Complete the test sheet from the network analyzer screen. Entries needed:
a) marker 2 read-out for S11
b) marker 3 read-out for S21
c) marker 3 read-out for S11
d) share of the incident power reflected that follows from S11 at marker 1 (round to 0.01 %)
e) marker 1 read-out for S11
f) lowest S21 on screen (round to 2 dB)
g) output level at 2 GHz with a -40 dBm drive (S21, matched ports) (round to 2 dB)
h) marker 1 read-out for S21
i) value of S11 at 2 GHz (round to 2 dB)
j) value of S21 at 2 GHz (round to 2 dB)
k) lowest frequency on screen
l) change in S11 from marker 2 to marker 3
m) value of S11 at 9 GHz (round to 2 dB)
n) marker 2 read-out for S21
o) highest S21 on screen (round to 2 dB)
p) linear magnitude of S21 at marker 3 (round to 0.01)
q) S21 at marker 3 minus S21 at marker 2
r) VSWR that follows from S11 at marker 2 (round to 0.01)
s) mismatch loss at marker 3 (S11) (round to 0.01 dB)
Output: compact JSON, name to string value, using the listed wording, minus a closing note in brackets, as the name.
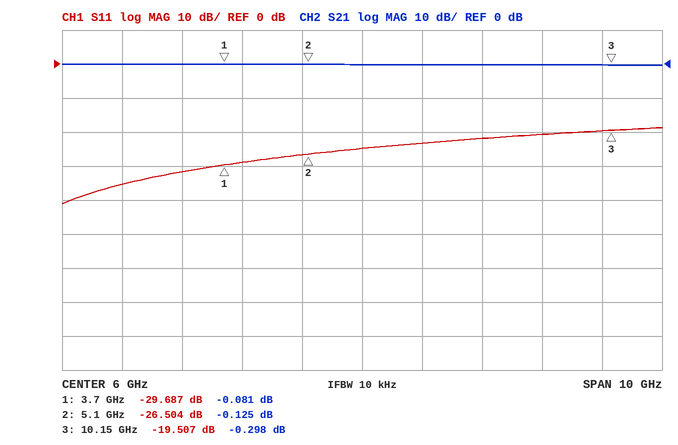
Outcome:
{"marker 2 read-out for S11": "-26.504 dB", "marker 3 read-out for S21": "-0.298 dB", "marker 3 read-out for S11": "-19.507 dB", "share of the incident power reflected that follows from S11 at marker 1": "0.11 %", "marker 1 read-out for S11": "-29.687 dB", "lowest S21 on screen": "0 dB", "output level at 2 GHz with a -40 dBm drive (S21, matched ports)": "-40 dBm", "marker 1 read-out for S21": "-0.081 dB", "value of S11 at 2 GHz": "-36 dB", "value of S21 at 2 GHz": "0 dB", "lowest frequency on screen": "1 GHz", "change in S11 from marker 2 to marker 3": "6.997 dB", "value of S11 at 9 GHz": "-20 dB", "marker 2 read-out for S21": "-0.125 dB", "highest S21 on screen": "0 dB", "linear magnitude of S21 at marker 3": "0.97", "S21 at marker 3 minus S21 at marker 2": "-0.173 dB", "VSWR that follows from S11 at marker 2": "1.10", "mismatch loss at marker 3 (S11)": "0.05 dB"}
